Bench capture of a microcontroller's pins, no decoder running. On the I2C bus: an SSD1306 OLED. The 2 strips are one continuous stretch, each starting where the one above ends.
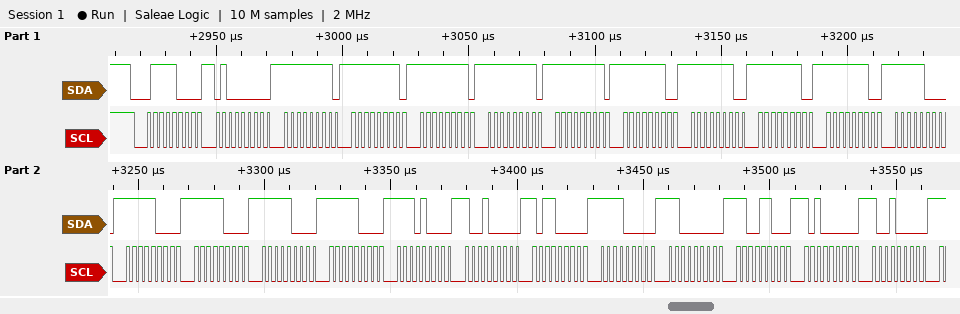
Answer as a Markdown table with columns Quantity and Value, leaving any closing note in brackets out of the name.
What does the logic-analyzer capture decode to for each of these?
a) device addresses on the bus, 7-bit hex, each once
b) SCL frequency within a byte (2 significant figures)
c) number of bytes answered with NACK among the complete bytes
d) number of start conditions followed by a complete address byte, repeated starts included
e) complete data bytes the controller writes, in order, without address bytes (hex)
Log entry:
| Quantity | Value |
|---|---|
| device addresses on the bus, 7-bit hex, each once | 0x3C |
| SCL frequency within a byte | 400 kHz |
| number of bytes answered with NACK among the complete bytes | 0 |
| number of start conditions followed by a complete address byte, repeated starts included | 1 |
| complete data bytes the controller writes, in order, without address bytes | 40 FF FF FF FF FF FE FE FE FE F8 F8 F8 F8 F8 E8 90 B0 F0 C0 CC A0 90 |
